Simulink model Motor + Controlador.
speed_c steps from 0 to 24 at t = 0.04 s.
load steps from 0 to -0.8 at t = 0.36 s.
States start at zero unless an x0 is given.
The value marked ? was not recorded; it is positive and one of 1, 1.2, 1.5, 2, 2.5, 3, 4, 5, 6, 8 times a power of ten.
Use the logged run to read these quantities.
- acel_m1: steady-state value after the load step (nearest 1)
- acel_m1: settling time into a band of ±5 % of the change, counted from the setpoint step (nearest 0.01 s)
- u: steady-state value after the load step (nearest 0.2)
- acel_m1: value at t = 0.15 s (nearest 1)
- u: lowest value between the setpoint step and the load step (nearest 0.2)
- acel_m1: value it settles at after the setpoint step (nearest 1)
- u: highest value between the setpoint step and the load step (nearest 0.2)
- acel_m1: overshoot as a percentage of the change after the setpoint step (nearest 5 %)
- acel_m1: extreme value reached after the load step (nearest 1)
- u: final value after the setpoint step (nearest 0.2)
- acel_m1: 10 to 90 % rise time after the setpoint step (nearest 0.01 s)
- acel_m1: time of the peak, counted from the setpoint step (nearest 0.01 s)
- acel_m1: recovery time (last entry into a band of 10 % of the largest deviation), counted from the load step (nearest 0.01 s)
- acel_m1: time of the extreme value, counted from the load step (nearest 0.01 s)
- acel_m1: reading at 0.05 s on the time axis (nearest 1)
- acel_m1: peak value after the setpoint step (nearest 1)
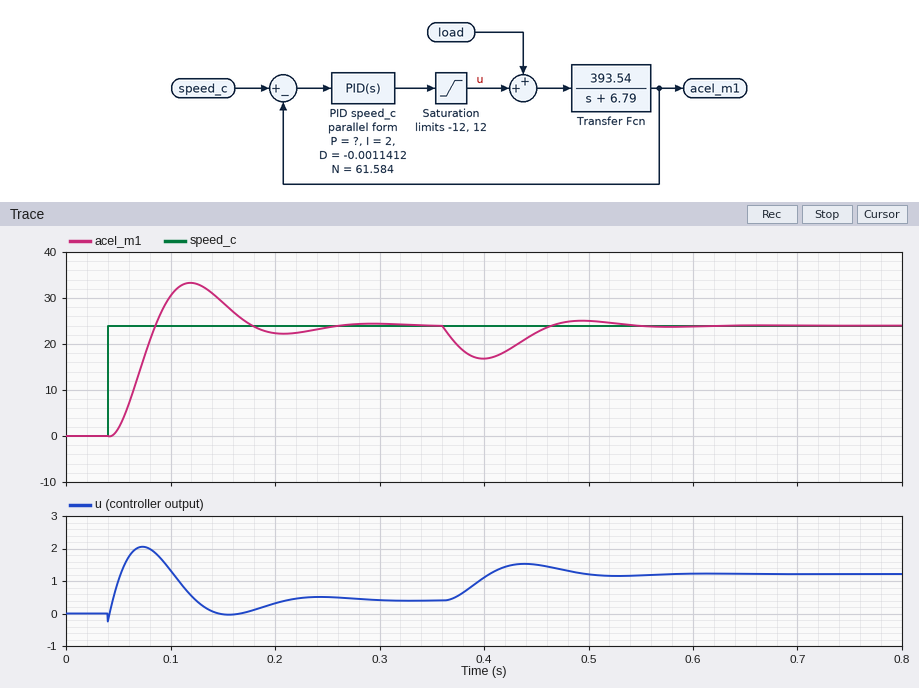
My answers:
24
0.19 s
1.2
29
-0.2
24
2.0
40 %
17
0.4
0.03 s
0.08 s
0.16 s
0.04 s
2
33
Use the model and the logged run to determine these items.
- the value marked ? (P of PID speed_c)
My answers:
0.06
